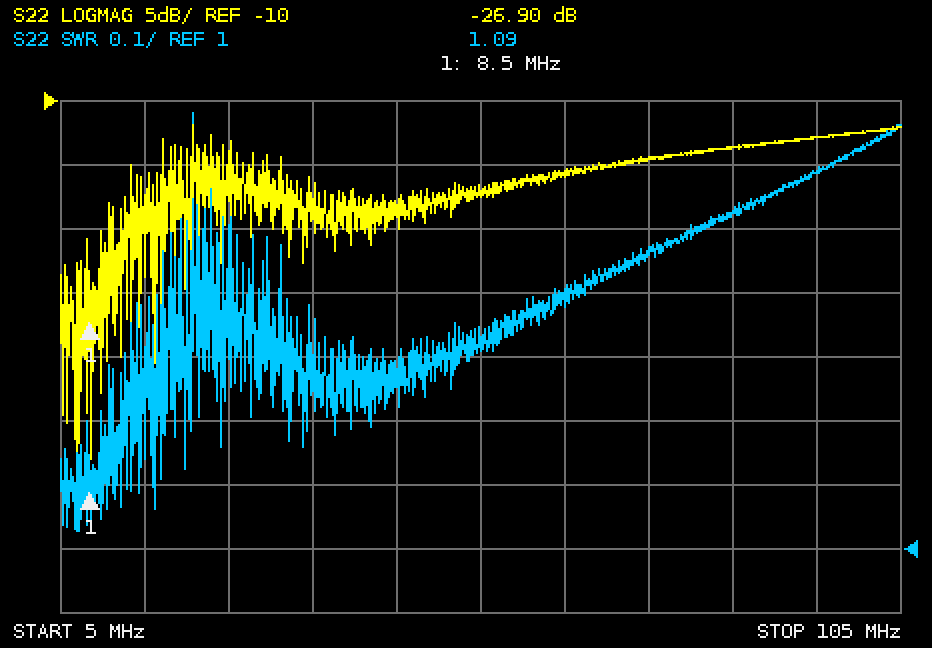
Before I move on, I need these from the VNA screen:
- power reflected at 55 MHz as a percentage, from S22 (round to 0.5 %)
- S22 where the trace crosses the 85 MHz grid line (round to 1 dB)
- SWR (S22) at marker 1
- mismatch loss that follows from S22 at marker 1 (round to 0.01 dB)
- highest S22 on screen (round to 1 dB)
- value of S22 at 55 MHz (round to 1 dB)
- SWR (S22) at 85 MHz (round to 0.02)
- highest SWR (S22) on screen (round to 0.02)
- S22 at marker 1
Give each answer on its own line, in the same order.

2.0 %
-14 dB
1.09
0.01 dB
-12 dB
-17 dB
1.52
1.68
-26.90 dB
